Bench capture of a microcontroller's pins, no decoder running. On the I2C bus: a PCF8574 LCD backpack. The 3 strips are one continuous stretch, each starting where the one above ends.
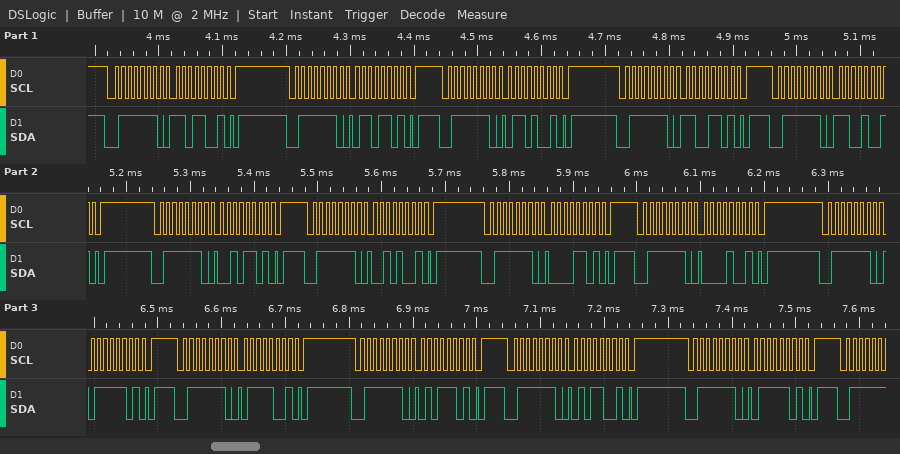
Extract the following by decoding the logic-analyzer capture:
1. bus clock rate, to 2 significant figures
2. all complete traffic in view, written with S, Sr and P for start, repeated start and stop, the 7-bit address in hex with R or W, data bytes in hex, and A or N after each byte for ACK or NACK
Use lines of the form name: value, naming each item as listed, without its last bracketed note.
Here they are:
bus clock rate, to 2 significant figures: 100 kHz
all complete traffic in view, written with S, Sr and P for start, repeated start and stop, the 7-bit address in hex with R or W, data bytes in hex, and A or N after each byte for ACK or NACK: S 3FW A D9 A P S 3FW A 6D A P S 3FW A 69 A P S 3FW A CD A P S 3FW A C9 A P S 3FW A 2D A P S 3FW A 29 A P S 3FW A 0D A P S 3FW A 09 A P S 3FW A 7D A P S 3FW A 79 A P S 3FW A 5D A P S 3FW A 59 A P S 3FW A 7D A P
